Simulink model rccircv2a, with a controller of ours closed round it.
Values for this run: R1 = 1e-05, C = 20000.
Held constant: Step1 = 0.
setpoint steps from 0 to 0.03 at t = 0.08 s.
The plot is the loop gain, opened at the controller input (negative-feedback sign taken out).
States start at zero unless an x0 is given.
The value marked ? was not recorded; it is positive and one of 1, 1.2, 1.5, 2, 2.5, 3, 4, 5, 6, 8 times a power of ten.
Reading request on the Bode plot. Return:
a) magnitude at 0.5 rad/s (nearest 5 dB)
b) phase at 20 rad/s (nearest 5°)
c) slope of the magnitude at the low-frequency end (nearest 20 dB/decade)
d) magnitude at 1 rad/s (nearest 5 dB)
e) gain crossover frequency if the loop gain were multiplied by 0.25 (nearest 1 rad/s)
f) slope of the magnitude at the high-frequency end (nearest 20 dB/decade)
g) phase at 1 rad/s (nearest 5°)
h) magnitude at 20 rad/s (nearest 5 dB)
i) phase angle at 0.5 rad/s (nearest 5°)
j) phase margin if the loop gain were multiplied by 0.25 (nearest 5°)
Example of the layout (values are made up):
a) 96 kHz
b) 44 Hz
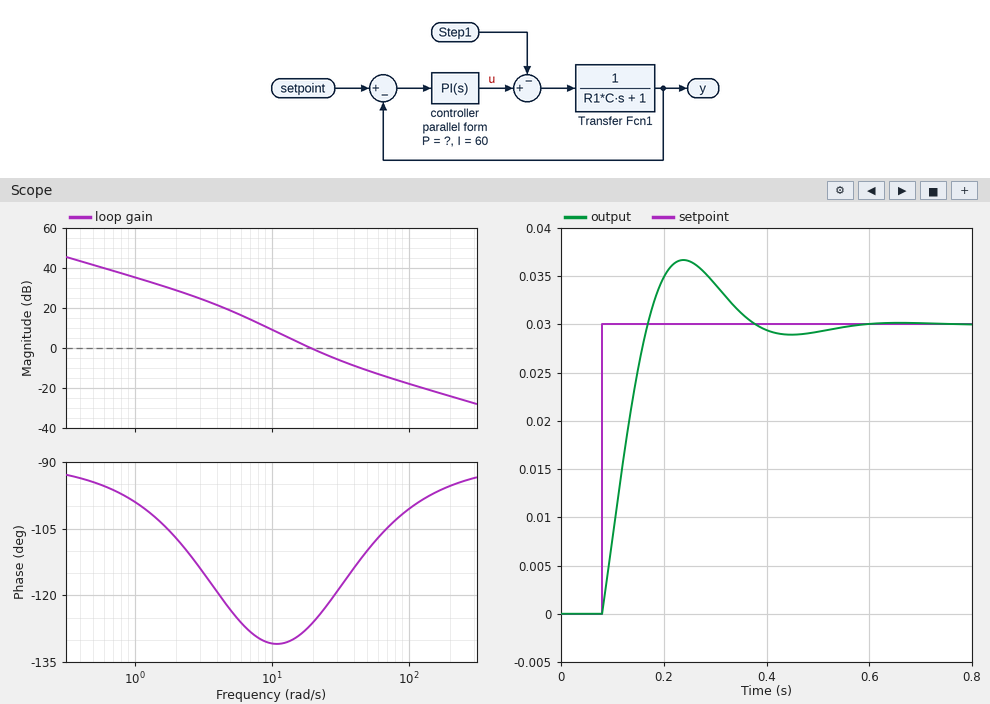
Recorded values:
a) 40 dB
b) -125°
c) -20 dB/decade
d) 35 dB
e) 8 rad/s
f) -20 dB/decade
g) -100°
h) 0 dB
i) -95°
j) 50°
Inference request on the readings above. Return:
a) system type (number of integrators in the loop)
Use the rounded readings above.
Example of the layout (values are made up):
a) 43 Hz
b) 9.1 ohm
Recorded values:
a) 1
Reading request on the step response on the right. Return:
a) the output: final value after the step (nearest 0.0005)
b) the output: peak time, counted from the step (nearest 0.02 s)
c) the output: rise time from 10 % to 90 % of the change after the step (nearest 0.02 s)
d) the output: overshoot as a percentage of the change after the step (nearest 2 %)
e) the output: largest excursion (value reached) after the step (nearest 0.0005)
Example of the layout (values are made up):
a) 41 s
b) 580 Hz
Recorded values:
a) 0.0300
b) 0.16 s
c) 0.06 s
d) 22 %
e) 0.0365
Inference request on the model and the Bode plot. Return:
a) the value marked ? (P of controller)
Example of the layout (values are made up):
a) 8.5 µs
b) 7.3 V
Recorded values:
a) 2.5
